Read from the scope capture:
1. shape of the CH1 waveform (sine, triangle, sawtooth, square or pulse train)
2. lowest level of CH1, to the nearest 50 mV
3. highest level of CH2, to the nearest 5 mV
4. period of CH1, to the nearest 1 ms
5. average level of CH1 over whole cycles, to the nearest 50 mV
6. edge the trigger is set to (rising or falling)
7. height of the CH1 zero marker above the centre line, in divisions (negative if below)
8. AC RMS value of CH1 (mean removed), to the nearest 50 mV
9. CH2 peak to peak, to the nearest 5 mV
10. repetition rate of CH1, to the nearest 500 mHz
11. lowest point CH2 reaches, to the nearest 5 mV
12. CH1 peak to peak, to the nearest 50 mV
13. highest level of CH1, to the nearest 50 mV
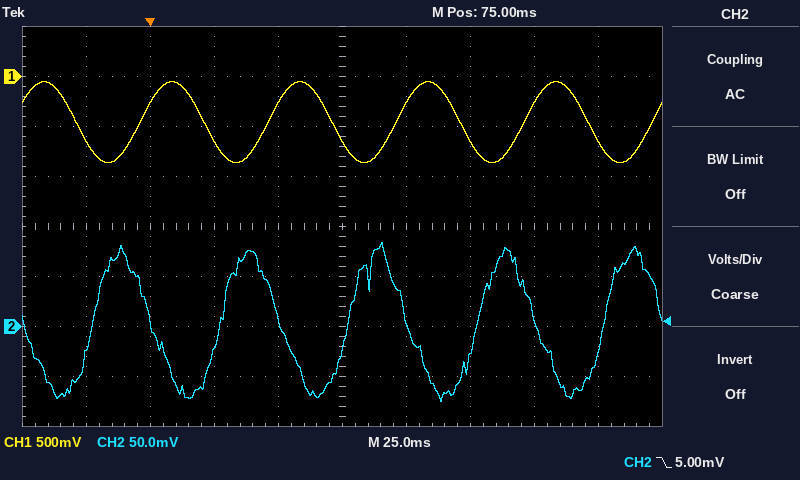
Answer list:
sine
-850 mV
85 mV
50 ms
-450 mV
falling
+3.0 div
300 mV
160 mV
20.0 Hz
-75 mV
800 mV
-50 mV
